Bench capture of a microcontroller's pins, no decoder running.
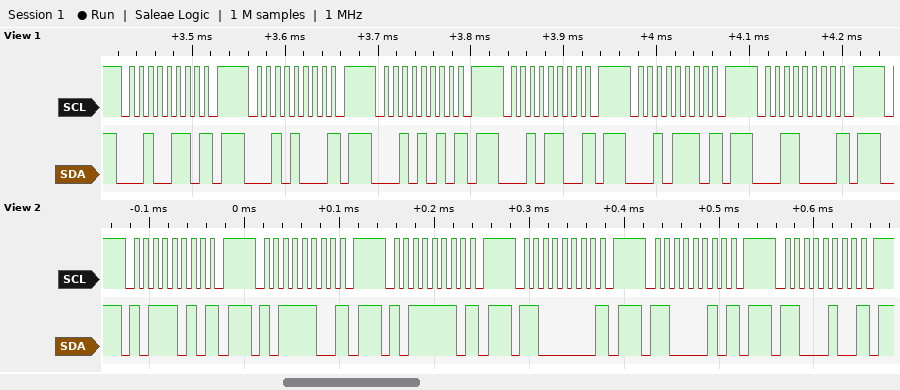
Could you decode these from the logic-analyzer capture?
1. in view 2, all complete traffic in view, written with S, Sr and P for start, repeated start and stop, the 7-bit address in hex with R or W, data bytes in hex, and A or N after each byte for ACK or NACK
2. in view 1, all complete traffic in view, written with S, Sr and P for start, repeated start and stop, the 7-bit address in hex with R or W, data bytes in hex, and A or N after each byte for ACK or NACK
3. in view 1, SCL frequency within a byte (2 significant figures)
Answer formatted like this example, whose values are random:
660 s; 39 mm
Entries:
S 5DW N P S 5EW N P S 5FW N P S 60W N P S 61W N P S 62W N P; S 13W N P S 14W N P S 15W N P S 16W N P S 17W N P S 18W N P; 100 kHz
